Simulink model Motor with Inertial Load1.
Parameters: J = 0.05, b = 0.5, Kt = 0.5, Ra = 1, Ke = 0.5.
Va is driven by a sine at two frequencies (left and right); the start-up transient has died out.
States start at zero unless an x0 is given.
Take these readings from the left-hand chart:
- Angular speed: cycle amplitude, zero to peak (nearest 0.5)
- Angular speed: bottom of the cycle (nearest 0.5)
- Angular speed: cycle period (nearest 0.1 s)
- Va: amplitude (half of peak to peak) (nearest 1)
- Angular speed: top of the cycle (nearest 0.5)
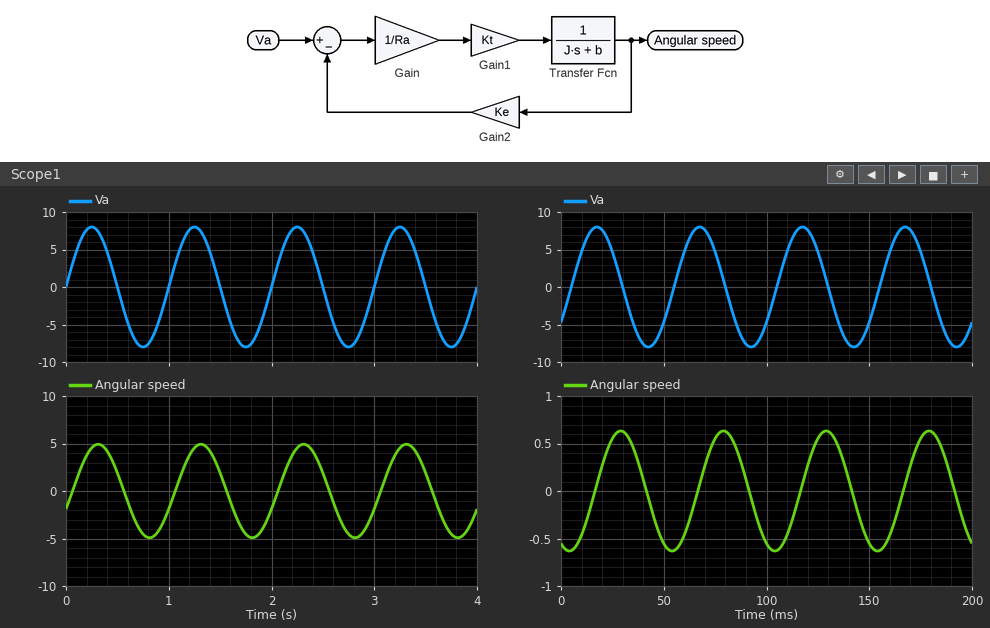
5.0
-5.0
1.0 s
8
5.0
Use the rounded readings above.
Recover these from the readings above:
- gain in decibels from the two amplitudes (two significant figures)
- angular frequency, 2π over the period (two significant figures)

-4.1 dB
6.3 rad/s
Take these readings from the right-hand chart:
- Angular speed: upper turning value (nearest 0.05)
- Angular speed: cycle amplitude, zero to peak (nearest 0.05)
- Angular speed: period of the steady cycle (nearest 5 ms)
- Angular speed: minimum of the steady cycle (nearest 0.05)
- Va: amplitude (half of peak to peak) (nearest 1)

0.65
0.65
50 ms
-0.65
8
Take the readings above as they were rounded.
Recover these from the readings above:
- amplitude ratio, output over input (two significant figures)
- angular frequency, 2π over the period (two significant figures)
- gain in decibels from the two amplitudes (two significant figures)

0.081
0.13 rad/ms
-22 dB
